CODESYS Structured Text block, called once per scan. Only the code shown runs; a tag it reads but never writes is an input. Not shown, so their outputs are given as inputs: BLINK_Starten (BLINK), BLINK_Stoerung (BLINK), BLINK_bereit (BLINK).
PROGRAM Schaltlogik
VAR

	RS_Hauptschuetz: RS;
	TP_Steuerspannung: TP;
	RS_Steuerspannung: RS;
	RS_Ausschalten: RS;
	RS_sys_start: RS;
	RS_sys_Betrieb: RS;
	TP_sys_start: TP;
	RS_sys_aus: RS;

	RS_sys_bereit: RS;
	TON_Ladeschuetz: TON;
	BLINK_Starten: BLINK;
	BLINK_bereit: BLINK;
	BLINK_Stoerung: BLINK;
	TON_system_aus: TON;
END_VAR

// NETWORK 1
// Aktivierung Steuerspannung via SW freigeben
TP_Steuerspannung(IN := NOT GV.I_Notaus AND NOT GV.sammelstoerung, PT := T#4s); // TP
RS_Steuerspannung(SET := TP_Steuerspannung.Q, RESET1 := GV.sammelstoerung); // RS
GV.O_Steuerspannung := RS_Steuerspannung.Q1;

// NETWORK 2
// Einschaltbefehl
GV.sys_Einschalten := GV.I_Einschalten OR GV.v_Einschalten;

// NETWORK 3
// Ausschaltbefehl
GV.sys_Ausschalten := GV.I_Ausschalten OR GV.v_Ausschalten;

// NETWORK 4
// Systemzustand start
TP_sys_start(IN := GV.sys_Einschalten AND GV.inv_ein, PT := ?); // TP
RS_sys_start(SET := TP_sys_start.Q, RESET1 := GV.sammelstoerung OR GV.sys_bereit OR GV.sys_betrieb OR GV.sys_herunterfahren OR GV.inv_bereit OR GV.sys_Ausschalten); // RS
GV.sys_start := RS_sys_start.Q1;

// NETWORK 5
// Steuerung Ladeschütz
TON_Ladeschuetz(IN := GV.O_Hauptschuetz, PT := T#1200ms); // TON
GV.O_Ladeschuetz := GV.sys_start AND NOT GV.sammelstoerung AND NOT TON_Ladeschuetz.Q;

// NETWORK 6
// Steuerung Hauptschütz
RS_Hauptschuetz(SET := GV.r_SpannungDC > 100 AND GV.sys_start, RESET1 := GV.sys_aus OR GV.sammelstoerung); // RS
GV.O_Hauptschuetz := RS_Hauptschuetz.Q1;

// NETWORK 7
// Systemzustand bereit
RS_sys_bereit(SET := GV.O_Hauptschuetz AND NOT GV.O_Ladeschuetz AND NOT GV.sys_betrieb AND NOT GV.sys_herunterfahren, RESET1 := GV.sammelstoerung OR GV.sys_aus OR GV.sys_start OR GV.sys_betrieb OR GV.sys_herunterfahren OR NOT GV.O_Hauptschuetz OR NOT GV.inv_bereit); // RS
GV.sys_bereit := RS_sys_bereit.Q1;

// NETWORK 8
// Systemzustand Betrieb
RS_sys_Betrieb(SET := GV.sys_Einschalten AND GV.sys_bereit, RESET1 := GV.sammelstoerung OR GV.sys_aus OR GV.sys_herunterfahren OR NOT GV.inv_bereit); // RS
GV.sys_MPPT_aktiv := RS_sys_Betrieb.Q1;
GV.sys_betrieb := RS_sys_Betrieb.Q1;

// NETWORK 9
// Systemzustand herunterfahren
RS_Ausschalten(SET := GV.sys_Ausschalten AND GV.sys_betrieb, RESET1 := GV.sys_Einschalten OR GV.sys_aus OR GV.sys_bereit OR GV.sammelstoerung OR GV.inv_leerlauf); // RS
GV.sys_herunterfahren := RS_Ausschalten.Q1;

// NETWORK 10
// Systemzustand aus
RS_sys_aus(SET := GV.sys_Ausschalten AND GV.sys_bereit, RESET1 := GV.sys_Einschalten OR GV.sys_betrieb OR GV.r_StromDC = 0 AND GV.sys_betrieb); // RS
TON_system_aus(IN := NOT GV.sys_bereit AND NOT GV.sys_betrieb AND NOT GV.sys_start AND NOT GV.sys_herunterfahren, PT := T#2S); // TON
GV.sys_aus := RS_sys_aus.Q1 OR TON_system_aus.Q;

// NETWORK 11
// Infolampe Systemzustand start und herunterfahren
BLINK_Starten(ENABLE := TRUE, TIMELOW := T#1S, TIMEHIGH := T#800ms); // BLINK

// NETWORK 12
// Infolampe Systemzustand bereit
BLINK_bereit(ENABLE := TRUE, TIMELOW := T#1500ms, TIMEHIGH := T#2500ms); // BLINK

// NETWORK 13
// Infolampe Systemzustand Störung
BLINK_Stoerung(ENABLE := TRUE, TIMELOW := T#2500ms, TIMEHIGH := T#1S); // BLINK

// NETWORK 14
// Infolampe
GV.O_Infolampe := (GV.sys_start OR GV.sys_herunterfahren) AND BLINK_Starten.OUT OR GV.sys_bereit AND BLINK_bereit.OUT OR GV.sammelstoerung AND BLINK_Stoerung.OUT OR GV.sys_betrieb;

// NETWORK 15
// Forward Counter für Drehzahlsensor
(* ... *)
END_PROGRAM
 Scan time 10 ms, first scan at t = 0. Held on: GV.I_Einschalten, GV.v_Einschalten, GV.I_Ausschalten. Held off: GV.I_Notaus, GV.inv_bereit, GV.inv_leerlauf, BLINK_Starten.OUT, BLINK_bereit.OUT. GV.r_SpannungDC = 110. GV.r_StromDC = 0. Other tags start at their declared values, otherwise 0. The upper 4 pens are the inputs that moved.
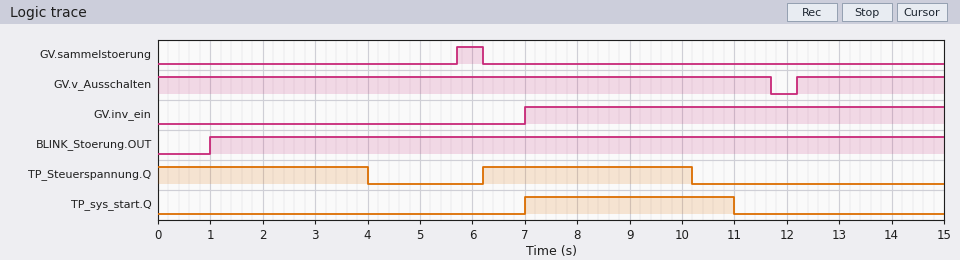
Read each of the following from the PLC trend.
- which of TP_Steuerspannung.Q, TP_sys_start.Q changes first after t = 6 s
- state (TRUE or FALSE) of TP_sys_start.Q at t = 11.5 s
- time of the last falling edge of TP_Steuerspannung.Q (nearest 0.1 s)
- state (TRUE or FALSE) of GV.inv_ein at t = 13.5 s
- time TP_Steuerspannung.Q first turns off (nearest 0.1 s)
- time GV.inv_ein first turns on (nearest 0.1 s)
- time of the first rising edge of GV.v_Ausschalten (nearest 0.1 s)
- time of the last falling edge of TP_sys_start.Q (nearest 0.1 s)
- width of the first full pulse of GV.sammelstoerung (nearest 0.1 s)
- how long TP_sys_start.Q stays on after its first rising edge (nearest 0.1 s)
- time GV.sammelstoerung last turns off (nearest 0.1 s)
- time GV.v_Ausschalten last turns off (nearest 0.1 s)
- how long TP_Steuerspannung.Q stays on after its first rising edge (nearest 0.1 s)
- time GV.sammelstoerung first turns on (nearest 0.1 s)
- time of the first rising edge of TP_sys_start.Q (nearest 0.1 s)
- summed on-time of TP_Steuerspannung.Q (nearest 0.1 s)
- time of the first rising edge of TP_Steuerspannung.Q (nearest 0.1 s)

TP_Steuerspannung.Q
FALSE
10.2 s
TRUE
4.0 s
7.0 s
12.2 s
11.0 s
0.5 s
4.0 s
6.2 s
11.7 s
4.0 s
5.7 s
7.0 s
8.0 s
6.2 s
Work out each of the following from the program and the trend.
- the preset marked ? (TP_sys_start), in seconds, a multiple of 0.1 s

4.0 s
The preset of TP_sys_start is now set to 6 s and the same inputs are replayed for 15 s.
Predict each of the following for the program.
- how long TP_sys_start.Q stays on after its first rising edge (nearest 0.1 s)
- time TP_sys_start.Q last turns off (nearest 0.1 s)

6.0 s
13.0 s
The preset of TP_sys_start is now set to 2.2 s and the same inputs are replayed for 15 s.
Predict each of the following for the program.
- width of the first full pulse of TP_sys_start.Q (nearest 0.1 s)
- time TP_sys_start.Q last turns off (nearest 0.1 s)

2.2 s
9.2 s
